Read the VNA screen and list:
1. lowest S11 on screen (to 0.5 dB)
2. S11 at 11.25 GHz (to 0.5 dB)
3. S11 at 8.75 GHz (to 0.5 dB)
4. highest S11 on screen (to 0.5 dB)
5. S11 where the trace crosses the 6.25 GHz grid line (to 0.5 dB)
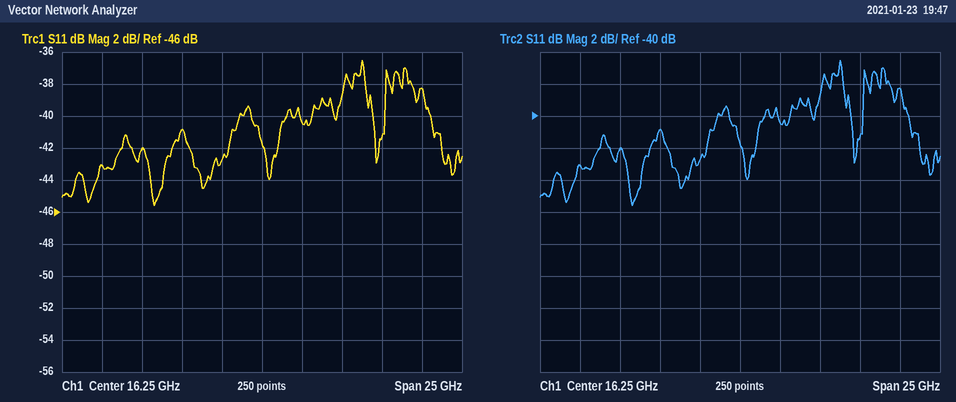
-45.5 dB
-41.0 dB
-42.0 dB
-36.5 dB
-43.0 dB
